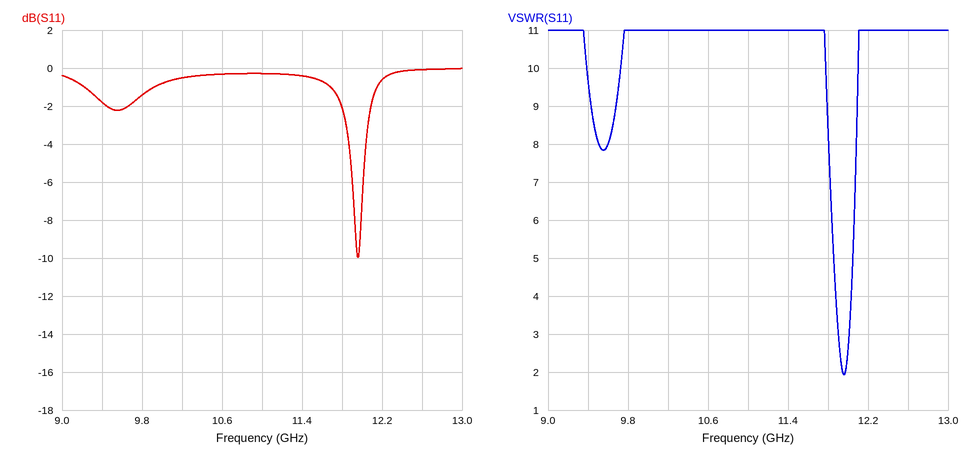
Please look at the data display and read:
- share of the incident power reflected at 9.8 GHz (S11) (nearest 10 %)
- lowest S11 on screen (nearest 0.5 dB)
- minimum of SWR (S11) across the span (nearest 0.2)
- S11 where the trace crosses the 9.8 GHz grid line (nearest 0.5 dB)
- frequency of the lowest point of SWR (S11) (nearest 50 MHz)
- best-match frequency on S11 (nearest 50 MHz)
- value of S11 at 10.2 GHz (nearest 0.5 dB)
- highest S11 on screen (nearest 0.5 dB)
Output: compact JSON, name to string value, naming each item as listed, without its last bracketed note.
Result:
{"share of the incident power reflected at 9.8 GHz (S11)": "70 %", "lowest S11 on screen": "-10.0 dB", "minimum of SWR (S11) across the span": "2.0", "S11 where the trace crosses the 9.8 GHz grid line": "-1.5 dB", "frequency of the lowest point of SWR (S11)": "11.95 GHz", "best-match frequency on S11": "11.95 GHz", "value of S11 at 10.2 GHz": "-0.5 dB", "highest S11 on screen": "0.0 dB"}
